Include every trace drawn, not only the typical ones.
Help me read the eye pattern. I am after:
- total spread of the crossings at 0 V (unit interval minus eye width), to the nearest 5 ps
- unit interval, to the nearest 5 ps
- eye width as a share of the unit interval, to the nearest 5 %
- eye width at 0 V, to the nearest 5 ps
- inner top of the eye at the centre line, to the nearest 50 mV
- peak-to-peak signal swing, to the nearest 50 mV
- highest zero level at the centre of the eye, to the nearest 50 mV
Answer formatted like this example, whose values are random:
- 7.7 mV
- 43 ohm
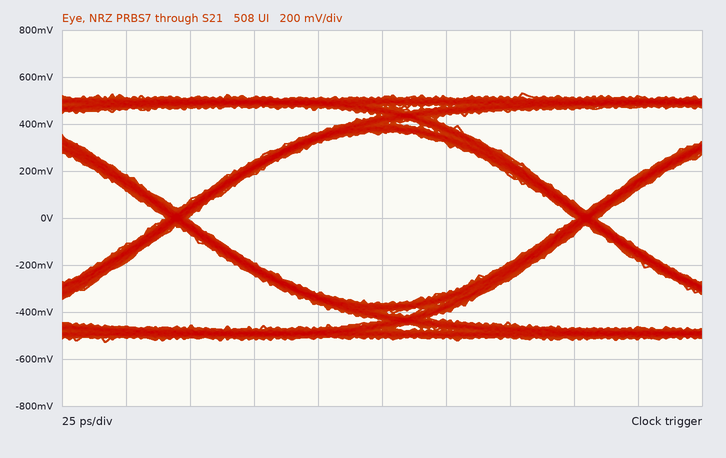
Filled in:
- 10 ps
- 160 ps
- 95 %
- 150 ps
- 350 mV
- 1.05 V
- -350 mV
